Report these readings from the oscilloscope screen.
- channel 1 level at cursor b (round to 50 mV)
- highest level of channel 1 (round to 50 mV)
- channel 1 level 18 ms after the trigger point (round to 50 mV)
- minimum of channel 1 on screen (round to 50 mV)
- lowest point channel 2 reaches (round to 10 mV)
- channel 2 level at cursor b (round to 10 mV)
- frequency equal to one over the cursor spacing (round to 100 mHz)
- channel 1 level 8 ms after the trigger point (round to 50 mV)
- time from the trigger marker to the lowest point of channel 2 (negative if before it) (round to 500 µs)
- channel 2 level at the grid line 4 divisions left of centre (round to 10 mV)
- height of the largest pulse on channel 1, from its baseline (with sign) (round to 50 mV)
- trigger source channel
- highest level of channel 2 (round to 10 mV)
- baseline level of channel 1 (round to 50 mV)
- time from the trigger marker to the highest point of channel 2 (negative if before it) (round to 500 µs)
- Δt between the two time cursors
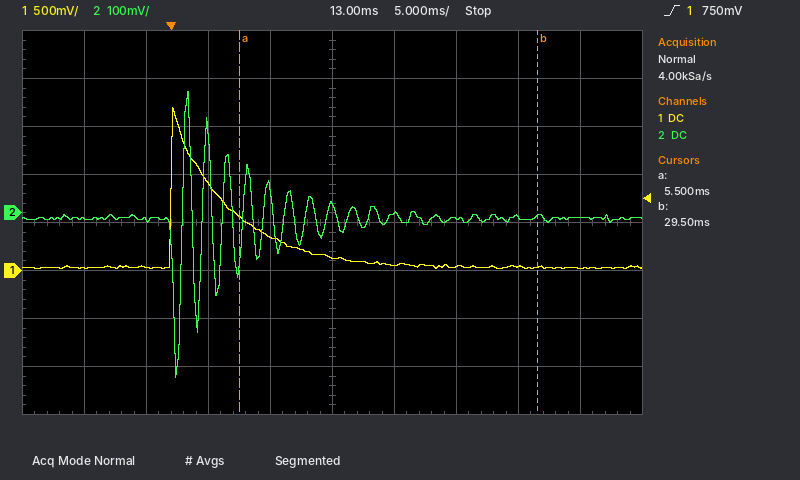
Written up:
50 mV
1.70 V
50 mV
0 mV
-340 mV
-10 mV
41.7 Hz
350 mV
+500 µs
-10 mV
+1.65 V
channel 1
250 mV
50 mV
+1.5 ms
24.0 ms
